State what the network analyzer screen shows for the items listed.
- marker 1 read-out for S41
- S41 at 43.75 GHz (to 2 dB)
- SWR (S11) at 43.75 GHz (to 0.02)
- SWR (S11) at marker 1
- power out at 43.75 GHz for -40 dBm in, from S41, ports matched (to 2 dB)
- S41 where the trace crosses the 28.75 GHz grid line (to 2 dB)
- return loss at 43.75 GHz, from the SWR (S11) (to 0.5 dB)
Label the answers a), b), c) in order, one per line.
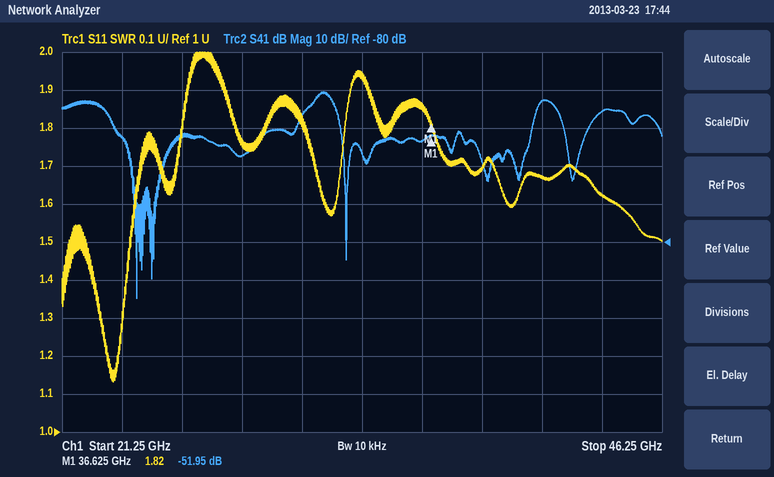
a) -51.95 dB
b) -46 dB
c) 1.62
d) 1.82
e) -86 dBm
f) -58 dB
g) 12.5 dB
